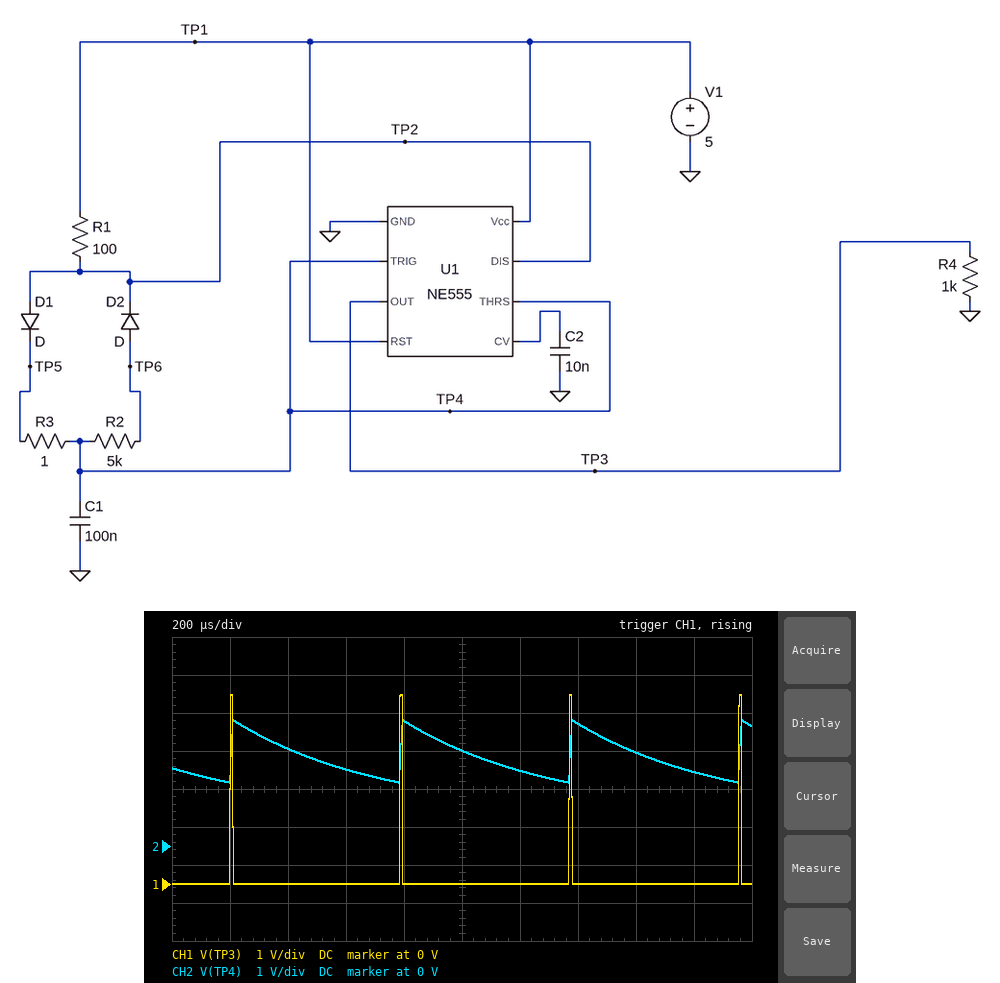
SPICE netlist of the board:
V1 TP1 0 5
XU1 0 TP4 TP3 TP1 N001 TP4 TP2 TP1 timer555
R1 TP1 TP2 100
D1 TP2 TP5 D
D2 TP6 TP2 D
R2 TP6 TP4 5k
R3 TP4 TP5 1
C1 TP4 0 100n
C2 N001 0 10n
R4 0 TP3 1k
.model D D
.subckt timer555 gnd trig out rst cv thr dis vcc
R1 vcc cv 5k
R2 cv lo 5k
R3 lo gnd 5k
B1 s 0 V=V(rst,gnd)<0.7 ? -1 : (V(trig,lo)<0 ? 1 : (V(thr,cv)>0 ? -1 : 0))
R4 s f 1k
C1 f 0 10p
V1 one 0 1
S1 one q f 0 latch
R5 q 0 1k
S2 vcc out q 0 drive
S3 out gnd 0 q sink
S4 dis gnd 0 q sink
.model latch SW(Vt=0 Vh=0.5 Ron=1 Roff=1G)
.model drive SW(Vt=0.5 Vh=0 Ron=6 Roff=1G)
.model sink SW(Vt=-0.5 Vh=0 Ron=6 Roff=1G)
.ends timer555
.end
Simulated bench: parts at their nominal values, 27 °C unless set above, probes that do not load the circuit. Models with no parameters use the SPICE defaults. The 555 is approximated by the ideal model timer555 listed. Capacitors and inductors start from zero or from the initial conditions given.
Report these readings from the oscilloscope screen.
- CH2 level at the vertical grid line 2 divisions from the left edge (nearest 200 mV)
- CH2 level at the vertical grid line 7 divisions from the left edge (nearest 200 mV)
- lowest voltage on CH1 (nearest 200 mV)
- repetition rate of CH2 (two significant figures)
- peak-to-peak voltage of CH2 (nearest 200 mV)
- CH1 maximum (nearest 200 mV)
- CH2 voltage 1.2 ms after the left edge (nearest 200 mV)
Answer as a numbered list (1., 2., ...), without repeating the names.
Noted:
1. 2.6 V
2. 3.2 V
3. 0 V
4. 1.7 kHz
5. 1.6 V
6. 5.0 V
7. 2.0 V
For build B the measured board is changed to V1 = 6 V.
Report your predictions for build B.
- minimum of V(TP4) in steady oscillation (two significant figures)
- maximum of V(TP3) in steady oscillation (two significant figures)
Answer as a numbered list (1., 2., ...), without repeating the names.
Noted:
1. 2.0 V
2. 6.0 V
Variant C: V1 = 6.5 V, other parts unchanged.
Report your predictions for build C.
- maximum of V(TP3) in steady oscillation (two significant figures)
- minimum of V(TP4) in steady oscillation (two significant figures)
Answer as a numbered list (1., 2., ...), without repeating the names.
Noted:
1. 6.5 V
2. 2.2 V
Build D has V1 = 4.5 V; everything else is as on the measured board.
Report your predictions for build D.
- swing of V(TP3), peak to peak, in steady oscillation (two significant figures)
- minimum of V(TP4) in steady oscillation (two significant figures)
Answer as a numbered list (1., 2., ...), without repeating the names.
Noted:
1. 4.5 V
2. 1.5 V
